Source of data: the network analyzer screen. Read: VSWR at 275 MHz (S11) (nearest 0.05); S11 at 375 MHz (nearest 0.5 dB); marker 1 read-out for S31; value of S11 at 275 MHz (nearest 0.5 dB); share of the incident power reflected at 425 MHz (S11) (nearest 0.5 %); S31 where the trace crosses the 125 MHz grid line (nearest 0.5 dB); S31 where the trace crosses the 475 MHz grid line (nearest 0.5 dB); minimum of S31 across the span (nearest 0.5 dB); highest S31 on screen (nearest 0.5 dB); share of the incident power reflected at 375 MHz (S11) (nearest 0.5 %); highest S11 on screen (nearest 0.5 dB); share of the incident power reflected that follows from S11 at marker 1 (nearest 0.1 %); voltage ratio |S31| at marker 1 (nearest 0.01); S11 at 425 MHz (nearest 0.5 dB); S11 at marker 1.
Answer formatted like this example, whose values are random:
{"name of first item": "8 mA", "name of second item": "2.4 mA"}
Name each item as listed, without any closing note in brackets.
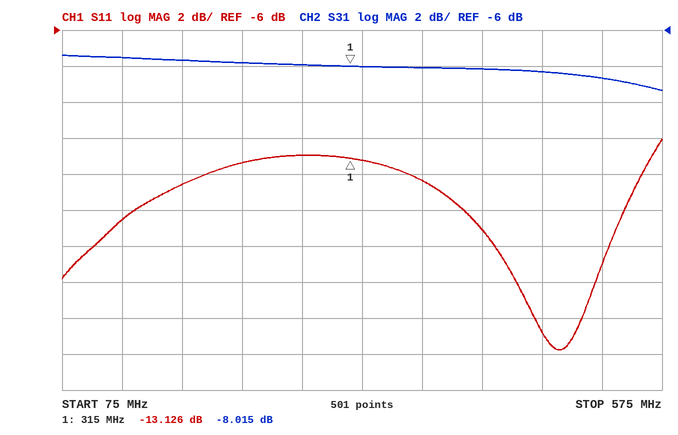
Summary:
{"VSWR at 275 MHz (S11)": "1.60", "S11 at 375 MHz": "-14.5 dB", "marker 1 read-out for S31": "-8.015 dB", "value of S11 at 275 MHz": "-13.0 dB", "share of the incident power reflected at 425 MHz (S11)": "2.0 %", "S31 where the trace crosses the 125 MHz grid line": "-7.5 dB", "S31 where the trace crosses the 475 MHz grid line": "-8.5 dB", "minimum of S31 across the span": "-9.5 dB", "highest S31 on screen": "-7.5 dB", "share of the incident power reflected at 375 MHz (S11)": "3.5 %", "highest S11 on screen": "-12.0 dB", "share of the incident power reflected that follows from S11 at marker 1": "4.9 %", "voltage ratio |S31| at marker 1": "0.40", "S11 at 425 MHz": "-17.0 dB", "S11 at marker 1": "-13.126 dB"}
